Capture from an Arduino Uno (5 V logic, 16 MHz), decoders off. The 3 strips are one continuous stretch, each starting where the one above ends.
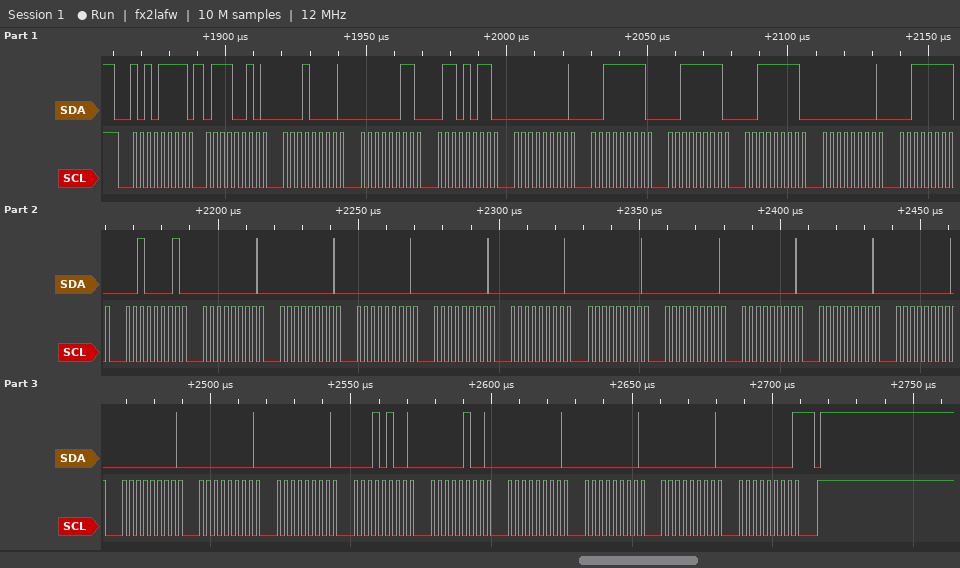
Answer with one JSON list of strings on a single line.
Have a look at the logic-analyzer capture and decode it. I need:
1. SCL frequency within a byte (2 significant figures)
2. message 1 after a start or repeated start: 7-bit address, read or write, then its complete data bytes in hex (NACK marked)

["400 kHz", "0x57 read: 72 10 03 6B 00 3F 3F 3F 00 3F 21 00 00 00 00 00 00 00 00 00 00 00 00 00 14 04 00 00 00 00 NACK"]
